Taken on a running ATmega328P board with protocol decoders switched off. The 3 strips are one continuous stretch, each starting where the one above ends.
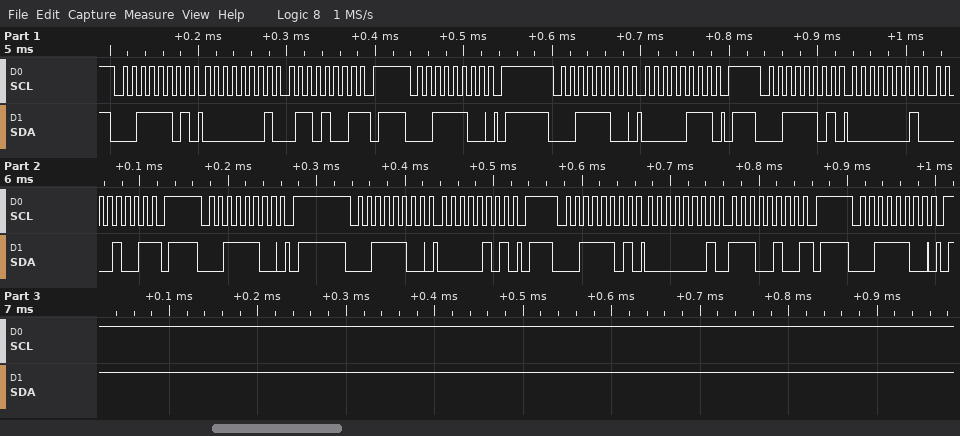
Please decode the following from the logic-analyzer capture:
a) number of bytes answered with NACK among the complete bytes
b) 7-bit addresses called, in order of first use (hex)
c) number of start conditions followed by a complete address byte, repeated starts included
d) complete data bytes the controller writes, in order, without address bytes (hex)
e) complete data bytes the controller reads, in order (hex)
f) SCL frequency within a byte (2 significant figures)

3
0x1E
8
07 05
01 69 01 09 01 E4
100 kHz
